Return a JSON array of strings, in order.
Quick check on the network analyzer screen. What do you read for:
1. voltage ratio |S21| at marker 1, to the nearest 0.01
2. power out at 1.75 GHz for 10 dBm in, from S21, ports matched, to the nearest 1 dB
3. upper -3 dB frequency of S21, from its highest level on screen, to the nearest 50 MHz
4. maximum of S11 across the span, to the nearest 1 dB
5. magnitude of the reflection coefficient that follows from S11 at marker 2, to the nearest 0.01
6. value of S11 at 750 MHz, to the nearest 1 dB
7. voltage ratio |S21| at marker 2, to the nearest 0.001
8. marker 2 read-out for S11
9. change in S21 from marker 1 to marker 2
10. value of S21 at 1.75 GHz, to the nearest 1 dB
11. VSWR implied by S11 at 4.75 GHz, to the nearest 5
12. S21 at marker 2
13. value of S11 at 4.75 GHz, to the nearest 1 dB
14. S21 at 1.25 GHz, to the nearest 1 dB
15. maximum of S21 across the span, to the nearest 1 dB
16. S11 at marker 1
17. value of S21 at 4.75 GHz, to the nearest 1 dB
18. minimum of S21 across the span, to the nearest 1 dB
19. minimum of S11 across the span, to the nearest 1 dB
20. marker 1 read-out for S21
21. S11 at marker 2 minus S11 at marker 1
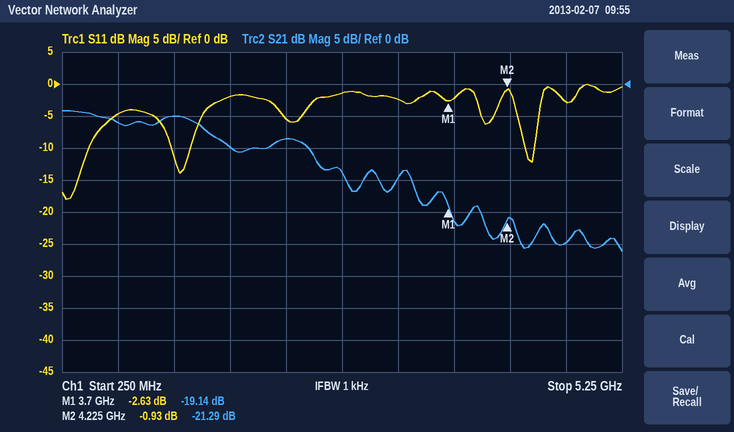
["0.11", "0 dBm", "1.55 GHz", "0 dB", "0.90", "-5 dB", "0.086", "-0.93 dB", "-2.15 dB", "-10 dB", "5", "-21.29 dB", "-3 dB", "-5 dB", "-4 dB", "-2.63 dB", "-25 dB", "-26 dB", "-18 dB", "-19.14 dB", "1.70 dB"]
